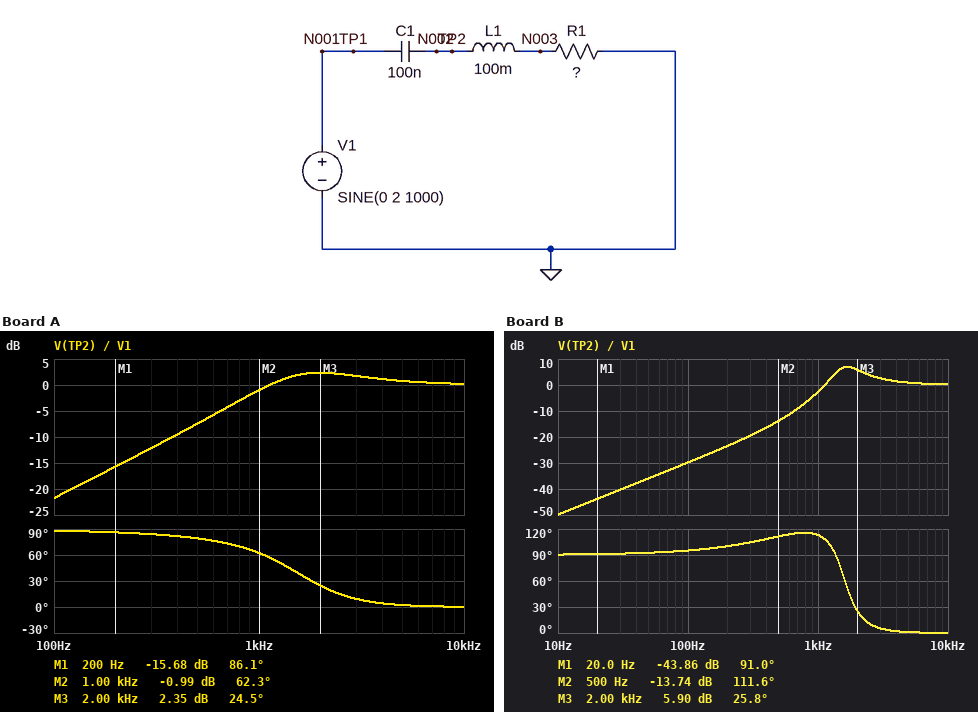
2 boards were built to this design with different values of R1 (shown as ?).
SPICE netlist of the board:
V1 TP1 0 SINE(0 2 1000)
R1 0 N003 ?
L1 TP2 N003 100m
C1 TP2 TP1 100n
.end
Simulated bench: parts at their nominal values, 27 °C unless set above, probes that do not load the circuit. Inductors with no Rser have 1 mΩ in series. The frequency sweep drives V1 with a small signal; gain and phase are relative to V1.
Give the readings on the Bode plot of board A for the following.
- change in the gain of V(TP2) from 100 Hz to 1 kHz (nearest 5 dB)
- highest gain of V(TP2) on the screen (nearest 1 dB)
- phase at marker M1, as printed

20 dB
2 dB
86.1 deg
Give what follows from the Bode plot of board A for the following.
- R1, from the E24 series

1.3 kΩ
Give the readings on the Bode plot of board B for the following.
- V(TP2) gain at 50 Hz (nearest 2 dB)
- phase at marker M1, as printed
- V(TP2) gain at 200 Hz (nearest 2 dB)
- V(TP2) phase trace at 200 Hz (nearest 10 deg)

-36 dB
91.0 deg
-24 dB
100 deg
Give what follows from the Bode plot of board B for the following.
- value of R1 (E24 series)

510 Ω
